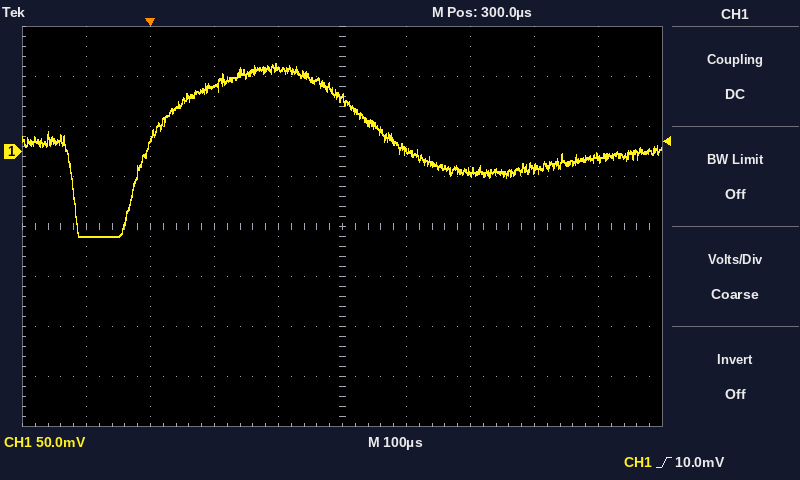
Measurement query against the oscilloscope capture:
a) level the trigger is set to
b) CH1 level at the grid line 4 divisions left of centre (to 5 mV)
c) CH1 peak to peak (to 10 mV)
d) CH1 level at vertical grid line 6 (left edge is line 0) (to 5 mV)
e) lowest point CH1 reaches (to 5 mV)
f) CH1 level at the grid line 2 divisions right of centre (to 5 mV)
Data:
10.0 mV
-85 mV
170 mV
0 mV
-85 mV
-20 mV
